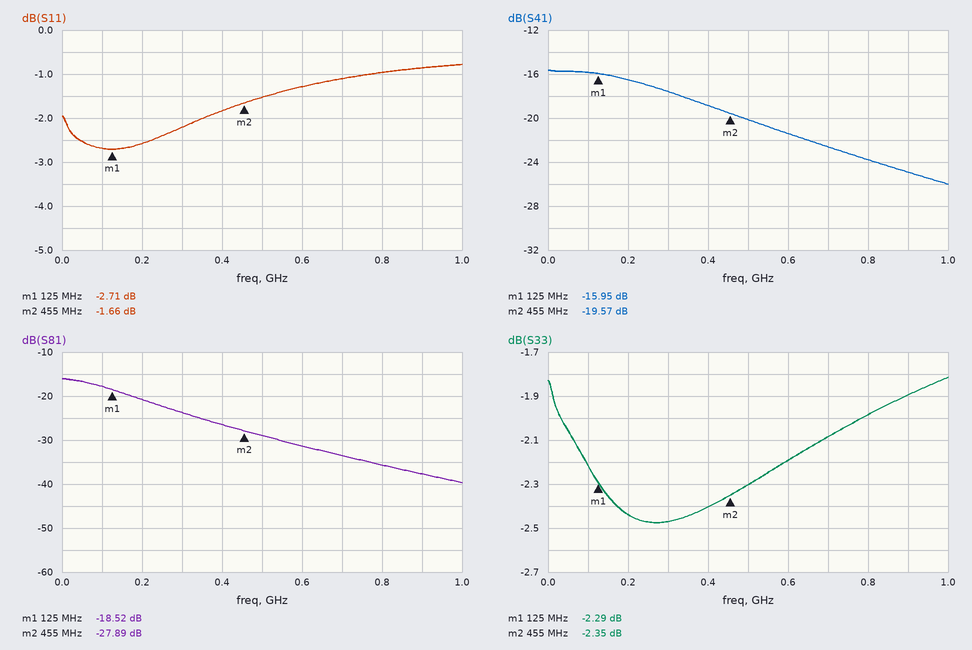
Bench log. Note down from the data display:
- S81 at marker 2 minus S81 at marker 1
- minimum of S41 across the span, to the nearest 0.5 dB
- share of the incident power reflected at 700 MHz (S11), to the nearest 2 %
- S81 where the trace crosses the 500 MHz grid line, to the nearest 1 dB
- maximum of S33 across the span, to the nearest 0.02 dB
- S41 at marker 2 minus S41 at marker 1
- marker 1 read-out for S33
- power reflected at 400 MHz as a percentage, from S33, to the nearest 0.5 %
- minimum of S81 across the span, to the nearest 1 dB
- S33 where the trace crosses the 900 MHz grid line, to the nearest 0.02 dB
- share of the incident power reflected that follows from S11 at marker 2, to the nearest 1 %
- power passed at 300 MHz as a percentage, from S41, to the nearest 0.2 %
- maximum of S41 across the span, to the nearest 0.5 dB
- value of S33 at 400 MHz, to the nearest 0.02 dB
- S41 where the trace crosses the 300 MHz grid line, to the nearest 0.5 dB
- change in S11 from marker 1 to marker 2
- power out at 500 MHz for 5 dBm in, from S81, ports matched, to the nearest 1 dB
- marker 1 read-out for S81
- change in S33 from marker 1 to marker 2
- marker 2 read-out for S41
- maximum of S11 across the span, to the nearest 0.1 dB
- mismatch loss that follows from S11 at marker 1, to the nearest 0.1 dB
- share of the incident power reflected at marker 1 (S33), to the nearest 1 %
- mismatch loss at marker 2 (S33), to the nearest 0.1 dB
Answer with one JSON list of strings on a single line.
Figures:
["-9.37 dB", "-26.0 dB", "78 %", "-29 dB", "-1.82 dB", "-3.62 dB", "-2.29 dB", "57.5 %", "-40 dB", "-1.90 dB", "68 %", "1.8 %", "-15.5 dB", "-2.40 dB", "-17.5 dB", "1.05 dB", "-24 dBm", "-18.52 dB", "-0.06 dB", "-19.57 dB", "-0.8 dB", "3.3 dB", "59 %", "3.8 dB"]
